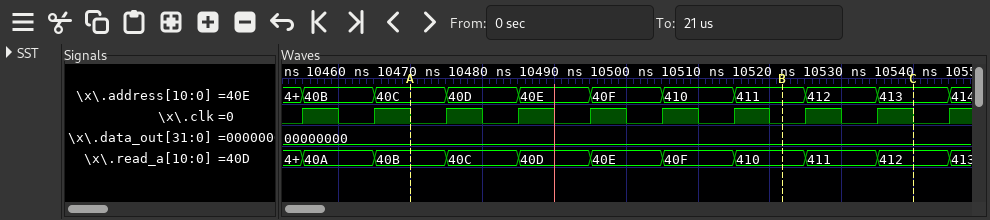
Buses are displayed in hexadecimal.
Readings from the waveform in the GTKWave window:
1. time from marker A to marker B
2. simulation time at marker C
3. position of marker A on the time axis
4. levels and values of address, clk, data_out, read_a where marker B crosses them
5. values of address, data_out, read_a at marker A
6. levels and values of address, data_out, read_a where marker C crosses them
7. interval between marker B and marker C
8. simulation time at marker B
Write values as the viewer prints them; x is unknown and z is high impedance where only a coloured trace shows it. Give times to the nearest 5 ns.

50 ns
10540 ns
10470 ns
address=411, clk=0, data_out=00000000, read_a=410
address=40C, data_out=00000000, read_a=40B
address=413, data_out=00000000, read_a=412
20 ns
10520 ns
